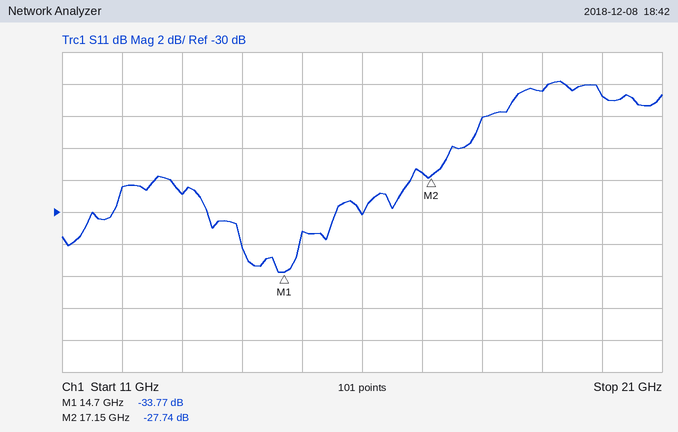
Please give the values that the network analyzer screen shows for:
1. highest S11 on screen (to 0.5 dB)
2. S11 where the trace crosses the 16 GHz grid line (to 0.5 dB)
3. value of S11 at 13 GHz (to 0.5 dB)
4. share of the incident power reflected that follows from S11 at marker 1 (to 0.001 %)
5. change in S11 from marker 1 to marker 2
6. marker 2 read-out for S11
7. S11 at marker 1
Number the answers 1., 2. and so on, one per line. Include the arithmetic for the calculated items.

1. -22.0 dB
2. -30.0 dB
3. -29.0 dB
4. 10^(-33.77/10) ≈ 0.042 %
5. -27.74 − (-33.77) = 6.03 dB
6. -27.74 dB
7. -33.77 dB
